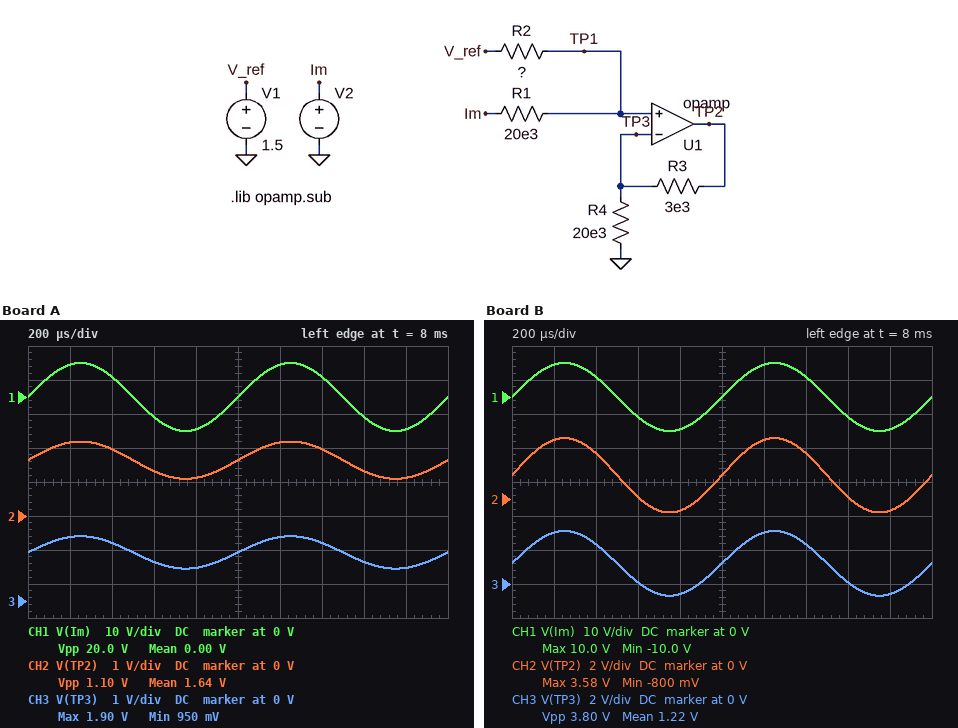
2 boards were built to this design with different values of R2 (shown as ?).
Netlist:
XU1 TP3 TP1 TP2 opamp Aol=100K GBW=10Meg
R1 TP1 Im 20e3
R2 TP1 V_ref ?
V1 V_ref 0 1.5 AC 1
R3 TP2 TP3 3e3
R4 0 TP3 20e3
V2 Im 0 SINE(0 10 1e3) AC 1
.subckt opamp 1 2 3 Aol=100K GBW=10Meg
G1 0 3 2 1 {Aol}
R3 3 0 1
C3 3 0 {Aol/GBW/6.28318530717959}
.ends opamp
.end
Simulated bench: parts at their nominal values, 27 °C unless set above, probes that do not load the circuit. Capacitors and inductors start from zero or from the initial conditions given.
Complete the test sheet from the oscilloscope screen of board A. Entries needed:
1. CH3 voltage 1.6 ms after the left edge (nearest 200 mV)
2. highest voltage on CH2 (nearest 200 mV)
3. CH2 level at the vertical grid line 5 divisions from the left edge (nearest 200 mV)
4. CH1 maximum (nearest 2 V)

1.2 V
2.2 V
1.6 V
10 V
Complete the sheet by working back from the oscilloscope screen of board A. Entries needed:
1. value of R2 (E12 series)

1 kΩ
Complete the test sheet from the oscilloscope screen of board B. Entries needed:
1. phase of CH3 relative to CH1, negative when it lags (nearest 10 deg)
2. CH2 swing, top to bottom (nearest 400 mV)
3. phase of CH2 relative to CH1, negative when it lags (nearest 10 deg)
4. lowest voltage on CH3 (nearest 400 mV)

0 deg
4.4 V
0 deg
-800 mV
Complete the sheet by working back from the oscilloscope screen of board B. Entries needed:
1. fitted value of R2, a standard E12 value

4.7 kΩ
